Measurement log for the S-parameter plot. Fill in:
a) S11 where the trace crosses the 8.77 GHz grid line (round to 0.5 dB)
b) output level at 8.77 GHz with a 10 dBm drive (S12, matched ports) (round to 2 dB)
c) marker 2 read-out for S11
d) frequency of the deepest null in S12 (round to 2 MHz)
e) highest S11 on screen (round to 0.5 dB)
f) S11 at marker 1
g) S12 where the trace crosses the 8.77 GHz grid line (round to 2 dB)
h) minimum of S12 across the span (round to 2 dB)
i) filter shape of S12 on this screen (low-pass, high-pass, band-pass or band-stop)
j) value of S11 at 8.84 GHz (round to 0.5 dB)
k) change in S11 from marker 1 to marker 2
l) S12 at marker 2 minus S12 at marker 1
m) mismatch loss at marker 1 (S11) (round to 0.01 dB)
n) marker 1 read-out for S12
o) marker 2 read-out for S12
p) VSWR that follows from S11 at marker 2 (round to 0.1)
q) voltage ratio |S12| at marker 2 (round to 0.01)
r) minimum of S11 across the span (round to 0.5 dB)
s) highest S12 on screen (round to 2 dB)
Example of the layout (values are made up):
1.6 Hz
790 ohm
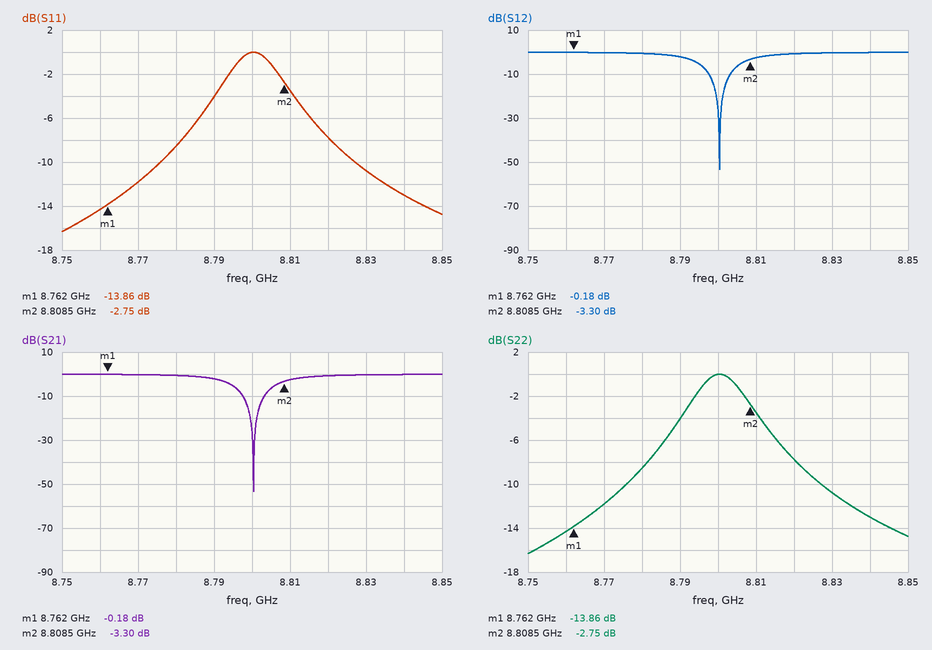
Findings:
-12.0 dB
10 dBm
-2.75 dB
8.800 GHz
0.0 dB
-13.86 dB
0 dB
-54 dB
band-stop
-13.0 dB
11.11 dB
-3.12 dB
0.18 dB
-0.18 dB
-3.30 dB
6.4
0.68
-16.5 dB
0 dB
